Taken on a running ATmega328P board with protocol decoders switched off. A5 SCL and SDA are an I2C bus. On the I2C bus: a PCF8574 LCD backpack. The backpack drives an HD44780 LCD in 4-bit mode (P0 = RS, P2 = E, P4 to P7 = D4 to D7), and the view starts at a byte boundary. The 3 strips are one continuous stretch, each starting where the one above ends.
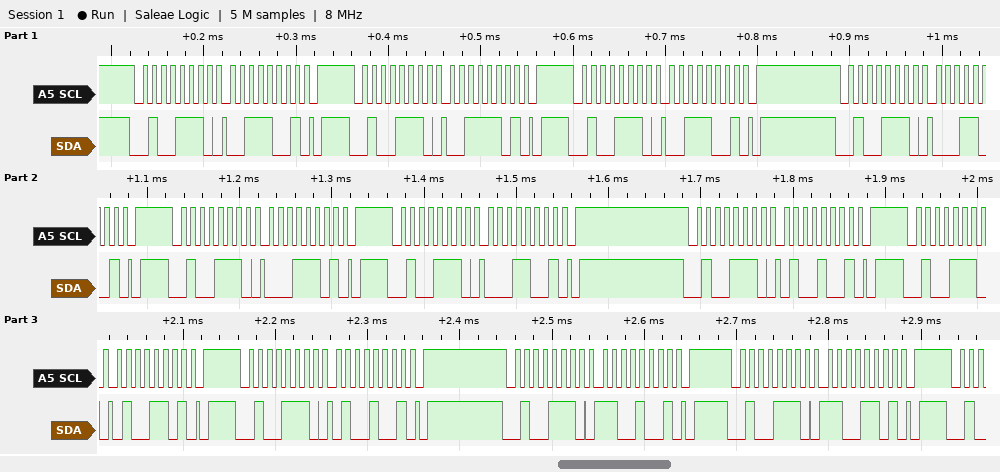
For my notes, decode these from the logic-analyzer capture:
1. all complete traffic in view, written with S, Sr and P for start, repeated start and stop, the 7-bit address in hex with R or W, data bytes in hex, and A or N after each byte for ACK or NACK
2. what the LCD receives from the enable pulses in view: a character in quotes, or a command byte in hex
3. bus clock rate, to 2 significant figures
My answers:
S 27W A 39 A P S 27W A 3D A P S 27W A 39 A P S 27W A 19 A P S 27W A 1D A P S 27W A 19 A P S 27W A 49 A P S 27W A 4D A P S 27W A 49 A P S 27W A C9 A P S 27W A CD A P
'1'
100 kHz
